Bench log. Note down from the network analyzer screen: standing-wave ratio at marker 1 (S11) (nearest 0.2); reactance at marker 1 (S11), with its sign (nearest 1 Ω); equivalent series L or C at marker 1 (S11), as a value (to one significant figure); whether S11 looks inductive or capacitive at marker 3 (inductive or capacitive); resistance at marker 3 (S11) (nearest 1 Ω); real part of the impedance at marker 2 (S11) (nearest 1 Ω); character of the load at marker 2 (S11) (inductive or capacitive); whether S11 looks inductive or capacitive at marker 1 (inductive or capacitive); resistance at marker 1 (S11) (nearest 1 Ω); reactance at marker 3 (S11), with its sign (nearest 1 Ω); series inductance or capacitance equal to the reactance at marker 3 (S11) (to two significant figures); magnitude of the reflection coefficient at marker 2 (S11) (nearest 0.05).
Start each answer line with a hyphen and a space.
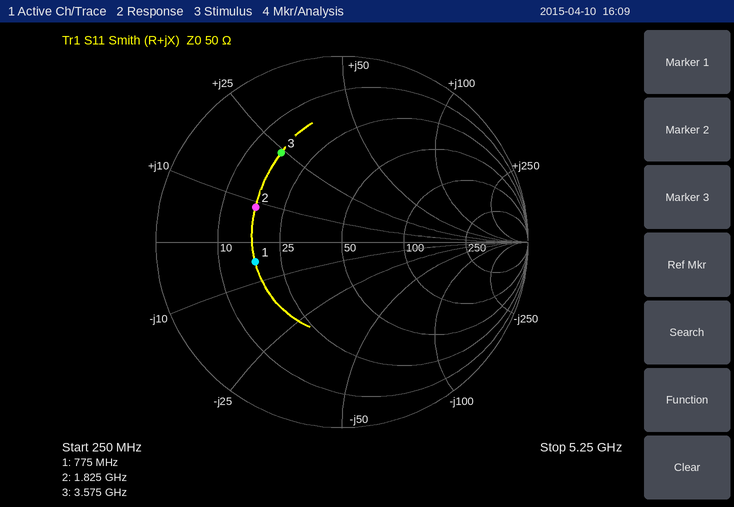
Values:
- 2.8
- -5 Ω
- 40 pF
- inductive
- 17 Ω
- 17 Ω
- inductive
- capacitive
- 18 Ω
- +24 Ω
- 1.1 nH
- 0.50
